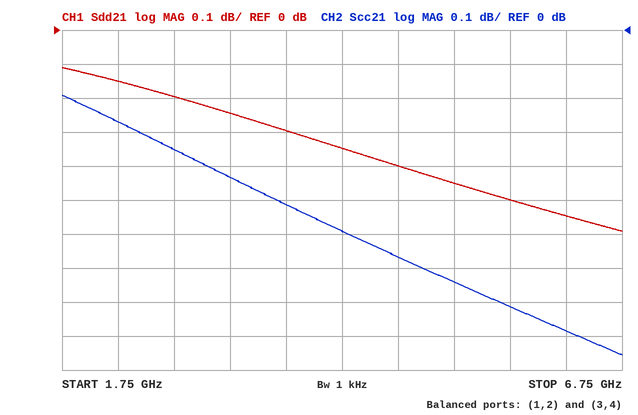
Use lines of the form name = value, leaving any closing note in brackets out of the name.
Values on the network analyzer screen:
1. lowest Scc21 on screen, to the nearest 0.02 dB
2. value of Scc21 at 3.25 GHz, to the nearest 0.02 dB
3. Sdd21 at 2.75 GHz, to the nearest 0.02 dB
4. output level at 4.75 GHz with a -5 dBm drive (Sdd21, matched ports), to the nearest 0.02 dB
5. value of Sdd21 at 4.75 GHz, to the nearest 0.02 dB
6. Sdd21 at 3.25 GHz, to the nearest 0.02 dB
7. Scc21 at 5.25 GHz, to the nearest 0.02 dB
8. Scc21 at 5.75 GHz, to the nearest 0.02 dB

lowest Scc21 on screen, to the nearest 0.02 dB = -0.96 dB
value of Scc21 at 3.25 GHz, to the nearest 0.02 dB = -0.44 dB
Sdd21 at 2.75 GHz, to the nearest 0.02 dB = -0.20 dB
output level at 4.75 GHz with a -5 dBm drive (Sdd21, matched ports), to the nearest 0.02 dB = -5.40 dBm
value of Sdd21 at 4.75 GHz, to the nearest 0.02 dB = -0.40 dB
Sdd21 at 3.25 GHz, to the nearest 0.02 dB = -0.24 dB
Scc21 at 5.25 GHz, to the nearest 0.02 dB = -0.74 dB
Scc21 at 5.75 GHz, to the nearest 0.02 dB = -0.82 dB
